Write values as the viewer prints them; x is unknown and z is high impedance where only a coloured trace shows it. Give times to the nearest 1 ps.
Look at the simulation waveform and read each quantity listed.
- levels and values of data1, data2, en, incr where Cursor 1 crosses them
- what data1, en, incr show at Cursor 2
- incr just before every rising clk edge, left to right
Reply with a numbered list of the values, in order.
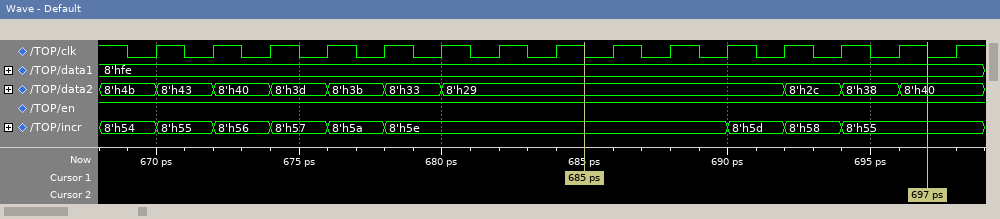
1. data1=8'hfe, data2=8'h29, en=1, incr=8'h5e
2. data1=8'hfe, en=1, incr=8'h55
3. 8'h54, 8'h55, 8'h56, 8'h57, 8'h5a, 8'h5e, 8'h5e, 8'h5e, 8'h5e, 8'h5e, 8'h5e, 8'h5d, 8'h58, 8'h55, 8'h55
